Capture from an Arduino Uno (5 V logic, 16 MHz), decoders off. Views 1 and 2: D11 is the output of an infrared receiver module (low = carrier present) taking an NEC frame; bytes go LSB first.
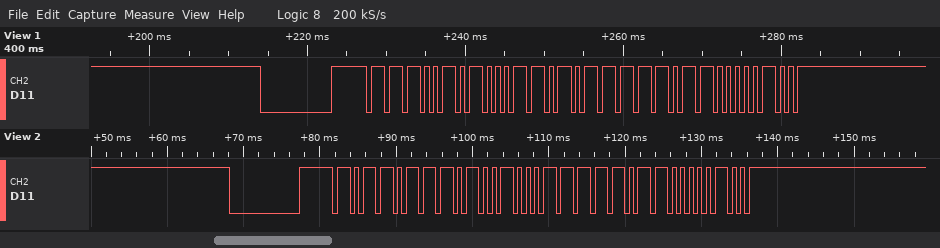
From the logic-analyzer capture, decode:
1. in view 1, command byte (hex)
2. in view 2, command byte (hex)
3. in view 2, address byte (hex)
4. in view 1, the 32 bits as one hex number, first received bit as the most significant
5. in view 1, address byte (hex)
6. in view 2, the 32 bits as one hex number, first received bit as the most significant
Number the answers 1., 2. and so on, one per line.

1. 0xDF
2. 0xDF
3. 0xED
4. 0xE51AFB04
5. 0xA7
6. 0xB748FB04
